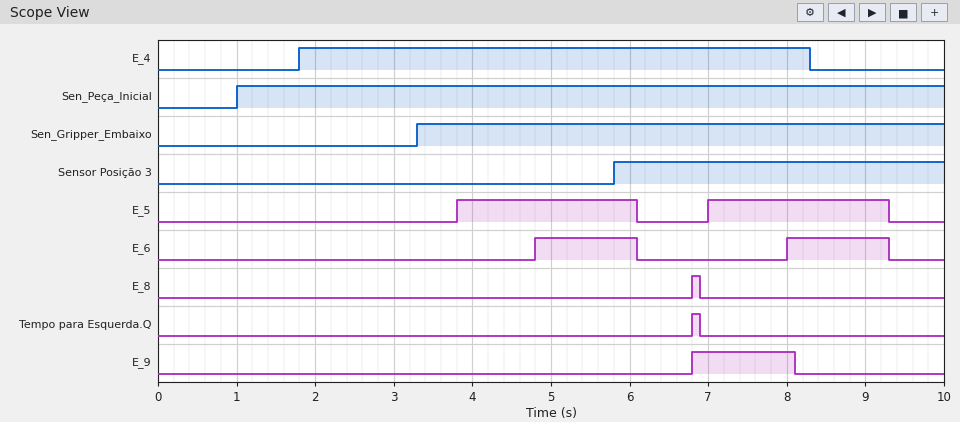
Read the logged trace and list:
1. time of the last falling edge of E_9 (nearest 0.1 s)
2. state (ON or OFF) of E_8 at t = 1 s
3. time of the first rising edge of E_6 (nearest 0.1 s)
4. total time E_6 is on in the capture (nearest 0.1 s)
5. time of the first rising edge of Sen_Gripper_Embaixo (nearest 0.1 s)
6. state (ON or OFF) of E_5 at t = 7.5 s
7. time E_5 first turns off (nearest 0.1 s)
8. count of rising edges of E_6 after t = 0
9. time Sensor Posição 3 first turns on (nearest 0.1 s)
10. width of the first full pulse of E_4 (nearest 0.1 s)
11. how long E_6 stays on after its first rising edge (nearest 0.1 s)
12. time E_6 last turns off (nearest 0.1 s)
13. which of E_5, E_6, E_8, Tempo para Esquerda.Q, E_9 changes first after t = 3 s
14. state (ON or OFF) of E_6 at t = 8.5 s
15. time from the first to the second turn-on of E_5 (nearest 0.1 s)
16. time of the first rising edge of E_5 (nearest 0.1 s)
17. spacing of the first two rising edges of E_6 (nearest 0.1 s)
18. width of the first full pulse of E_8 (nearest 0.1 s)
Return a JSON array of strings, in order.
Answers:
["8.1 s", "OFF", "4.8 s", "2.6 s", "3.3 s", "ON", "6.1 s", "2", "5.8 s", "6.5 s", "1.3 s", "9.3 s", "E_5", "ON", "3.2 s", "3.8 s", "3.2 s", "0.1 s"]
